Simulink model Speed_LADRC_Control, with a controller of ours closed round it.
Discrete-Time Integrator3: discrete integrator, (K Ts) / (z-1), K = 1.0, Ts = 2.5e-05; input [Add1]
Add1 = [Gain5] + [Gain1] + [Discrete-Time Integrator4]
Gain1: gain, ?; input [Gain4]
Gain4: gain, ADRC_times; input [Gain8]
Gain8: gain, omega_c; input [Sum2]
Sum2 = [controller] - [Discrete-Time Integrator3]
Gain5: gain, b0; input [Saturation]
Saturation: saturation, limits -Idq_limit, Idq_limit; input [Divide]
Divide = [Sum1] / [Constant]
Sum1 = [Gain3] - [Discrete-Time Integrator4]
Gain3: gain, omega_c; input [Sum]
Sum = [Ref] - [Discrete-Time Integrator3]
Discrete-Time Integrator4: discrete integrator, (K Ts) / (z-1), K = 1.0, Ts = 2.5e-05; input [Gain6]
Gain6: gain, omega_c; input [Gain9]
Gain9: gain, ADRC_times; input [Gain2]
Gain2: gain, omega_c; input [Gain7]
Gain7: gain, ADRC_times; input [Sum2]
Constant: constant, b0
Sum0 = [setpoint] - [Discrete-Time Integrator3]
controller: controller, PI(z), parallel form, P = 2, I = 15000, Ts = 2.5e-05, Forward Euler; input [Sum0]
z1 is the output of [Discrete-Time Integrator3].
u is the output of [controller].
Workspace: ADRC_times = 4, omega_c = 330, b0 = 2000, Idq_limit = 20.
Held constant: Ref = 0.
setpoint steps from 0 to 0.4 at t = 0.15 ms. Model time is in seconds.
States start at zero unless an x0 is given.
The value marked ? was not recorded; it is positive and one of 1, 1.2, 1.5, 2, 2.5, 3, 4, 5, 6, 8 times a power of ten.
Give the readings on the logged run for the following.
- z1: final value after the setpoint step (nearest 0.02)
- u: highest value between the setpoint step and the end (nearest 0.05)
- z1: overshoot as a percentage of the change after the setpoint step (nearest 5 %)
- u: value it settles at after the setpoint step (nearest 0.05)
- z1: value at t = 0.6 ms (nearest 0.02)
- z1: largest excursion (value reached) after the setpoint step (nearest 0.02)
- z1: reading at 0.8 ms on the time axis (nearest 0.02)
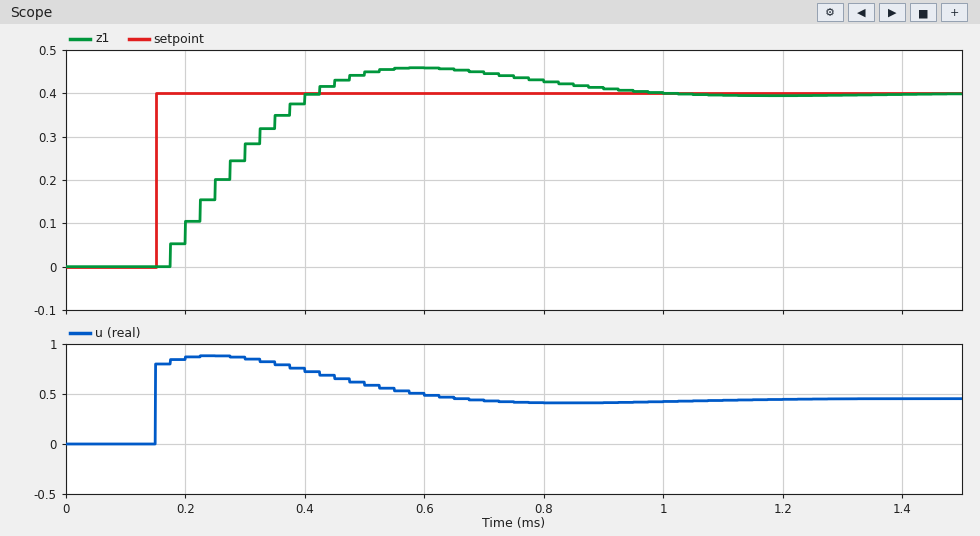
0.40
0.90
15 %
0.45
0.46
0.46
0.42
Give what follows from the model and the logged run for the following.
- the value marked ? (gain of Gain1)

2
